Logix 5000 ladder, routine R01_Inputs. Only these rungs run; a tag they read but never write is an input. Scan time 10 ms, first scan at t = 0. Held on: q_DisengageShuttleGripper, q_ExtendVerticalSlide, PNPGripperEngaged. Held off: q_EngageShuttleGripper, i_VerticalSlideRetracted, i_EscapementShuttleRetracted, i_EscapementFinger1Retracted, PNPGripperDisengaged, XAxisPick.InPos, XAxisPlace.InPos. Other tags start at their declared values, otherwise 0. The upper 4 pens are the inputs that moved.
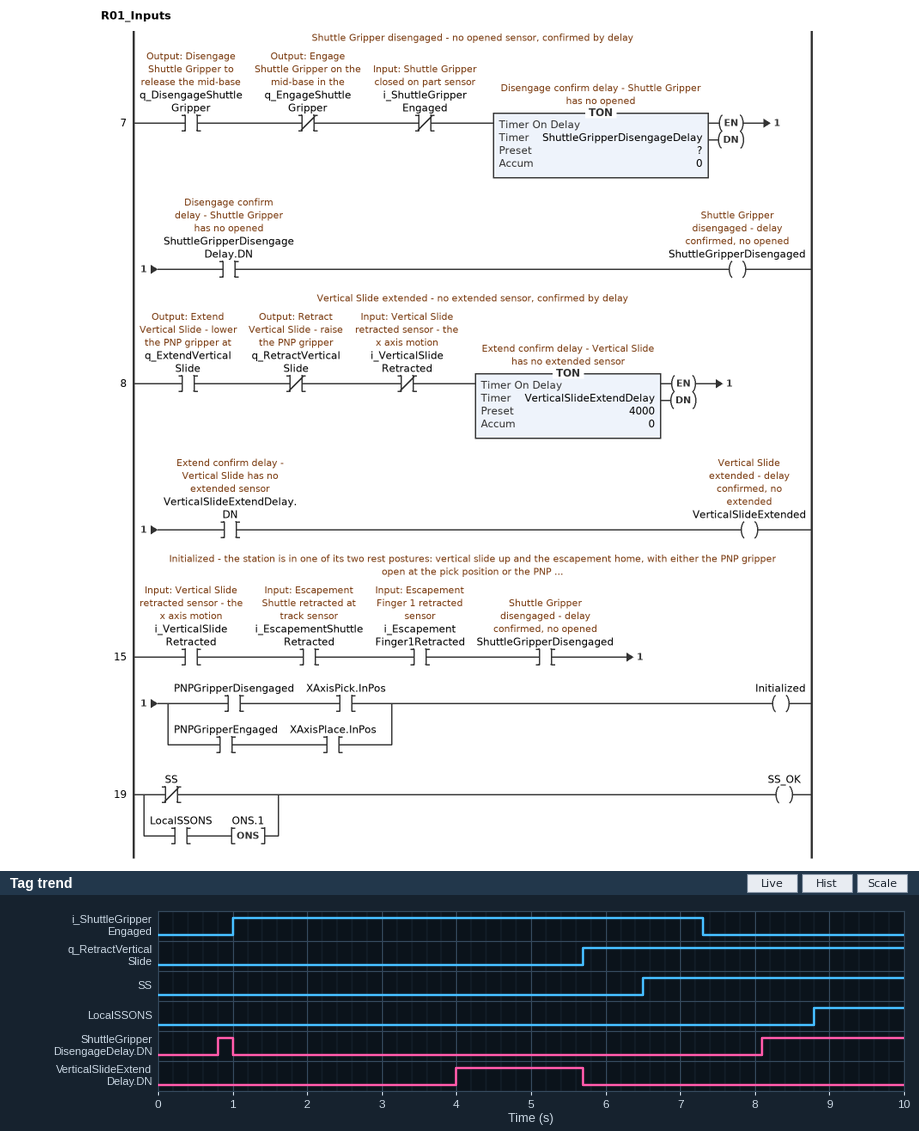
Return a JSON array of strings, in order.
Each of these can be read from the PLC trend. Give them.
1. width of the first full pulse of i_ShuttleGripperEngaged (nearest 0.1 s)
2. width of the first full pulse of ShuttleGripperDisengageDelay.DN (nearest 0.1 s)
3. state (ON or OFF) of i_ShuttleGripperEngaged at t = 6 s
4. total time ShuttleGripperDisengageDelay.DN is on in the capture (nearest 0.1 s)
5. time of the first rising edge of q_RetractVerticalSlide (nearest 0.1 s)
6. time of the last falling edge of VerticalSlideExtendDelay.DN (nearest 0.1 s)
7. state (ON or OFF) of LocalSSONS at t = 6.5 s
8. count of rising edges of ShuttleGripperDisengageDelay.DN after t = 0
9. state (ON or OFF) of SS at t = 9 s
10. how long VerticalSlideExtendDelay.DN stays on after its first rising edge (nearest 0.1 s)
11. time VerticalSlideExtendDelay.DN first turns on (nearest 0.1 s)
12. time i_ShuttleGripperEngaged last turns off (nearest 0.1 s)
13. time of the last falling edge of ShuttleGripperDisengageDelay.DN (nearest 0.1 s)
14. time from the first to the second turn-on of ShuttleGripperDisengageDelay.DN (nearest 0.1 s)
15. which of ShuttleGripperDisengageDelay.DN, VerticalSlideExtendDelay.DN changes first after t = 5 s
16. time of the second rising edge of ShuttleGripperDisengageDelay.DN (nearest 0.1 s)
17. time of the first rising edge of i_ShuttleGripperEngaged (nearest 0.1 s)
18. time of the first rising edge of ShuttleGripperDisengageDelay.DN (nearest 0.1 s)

["6.3 s", "0.2 s", "ON", "2.1 s", "5.7 s", "5.7 s", "OFF", "2", "ON", "1.7 s", "4.0 s", "7.3 s", "1.0 s", "7.3 s", "VerticalSlideExtendDelay.DN", "8.1 s", "1.0 s", "0.8 s"]
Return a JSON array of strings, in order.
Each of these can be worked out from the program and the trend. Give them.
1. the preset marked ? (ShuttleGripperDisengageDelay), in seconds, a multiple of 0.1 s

["0.8 s"]
